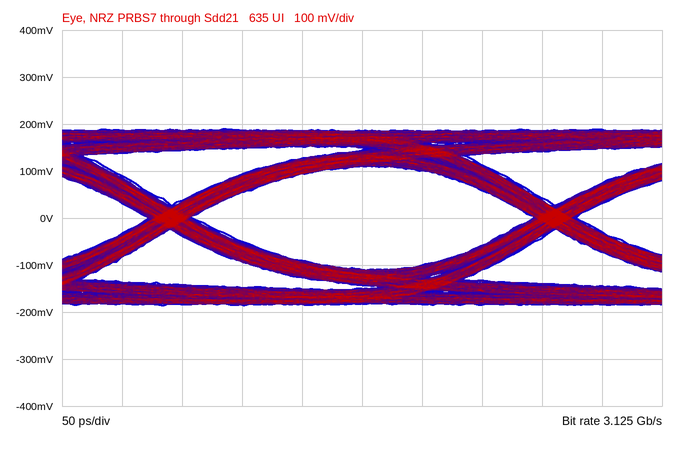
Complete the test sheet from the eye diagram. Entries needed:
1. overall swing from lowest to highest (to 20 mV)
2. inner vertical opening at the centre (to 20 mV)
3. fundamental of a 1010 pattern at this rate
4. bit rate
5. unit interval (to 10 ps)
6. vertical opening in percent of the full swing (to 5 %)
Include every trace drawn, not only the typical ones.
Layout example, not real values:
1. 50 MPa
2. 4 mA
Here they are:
1. 380 mV
2. 220 mV
3. 1.5625 GHz
4. 3.125 Gb/s
5. 320 ps
6. 60 %
